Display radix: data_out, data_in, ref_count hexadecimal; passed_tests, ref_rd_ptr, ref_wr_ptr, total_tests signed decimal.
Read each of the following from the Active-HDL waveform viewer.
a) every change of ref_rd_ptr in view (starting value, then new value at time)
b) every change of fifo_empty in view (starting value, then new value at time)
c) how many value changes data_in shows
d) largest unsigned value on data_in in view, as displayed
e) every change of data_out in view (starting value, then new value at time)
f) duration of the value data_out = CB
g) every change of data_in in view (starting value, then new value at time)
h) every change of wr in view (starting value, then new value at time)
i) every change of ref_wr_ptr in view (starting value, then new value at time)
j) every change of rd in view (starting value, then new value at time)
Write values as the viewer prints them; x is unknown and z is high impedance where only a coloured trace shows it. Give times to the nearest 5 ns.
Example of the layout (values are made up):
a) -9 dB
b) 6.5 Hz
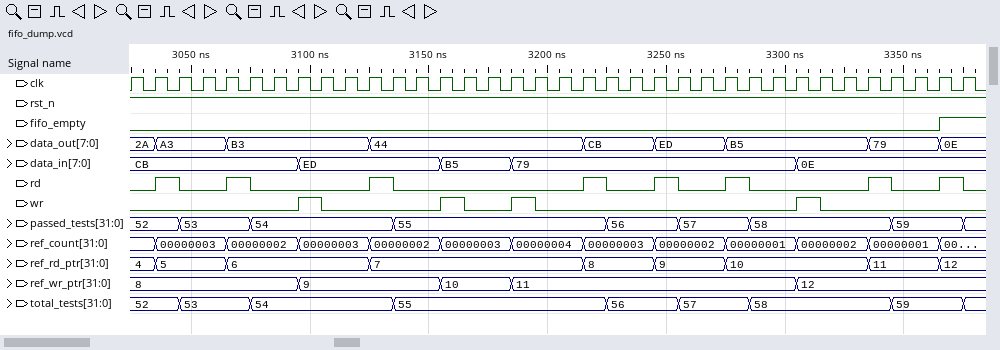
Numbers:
a) 4, 5 at 3035 ns, 6 at 3065 ns, 7 at 3125 ns, 8 at 3215 ns, 9 at 3245 ns, 10 at 3275 ns, 11 at 3335 ns, 12 at 3365 ns
b) 0, 1 at 3365 ns
c) 4
d) ED
e) 2A, A3 at 3035 ns, B3 at 3065 ns, 44 at 3125 ns, CB at 3215 ns, ED at 3245 ns, B5 at 3275 ns, 79 at 3335 ns, 0E at 3365 ns
f) 30 ns
g) CB, ED at 3095 ns, B5 at 3155 ns, 79 at 3185 ns, 0E at 3305 ns
h) 0, 1 at 3095 ns, 0 at 3105 ns, 1 at 3155 ns, 0 at 3165 ns, 1 at 3185 ns, 0 at 3195 ns, 1 at 3305 ns, 0 at 3315 ns
i) 8, 9 at 3095 ns, 10 at 3155 ns, 11 at 3185 ns, 12 at 3305 ns
j) 0, 1 at 3035 ns, 0 at 3045 ns, 1 at 3065 ns, 0 at 3075 ns, 1 at 3125 ns, 0 at 3135 ns, 1 at 3215 ns, 0 at 3225 ns, 1 at 3245 ns, 0 at 3255 ns, 1 at 3275 ns, 0 at 3285 ns, 1 at 3335 ns, 0 at 3345 ns, 1 at 3365 ns, 0 at 3375 ns
